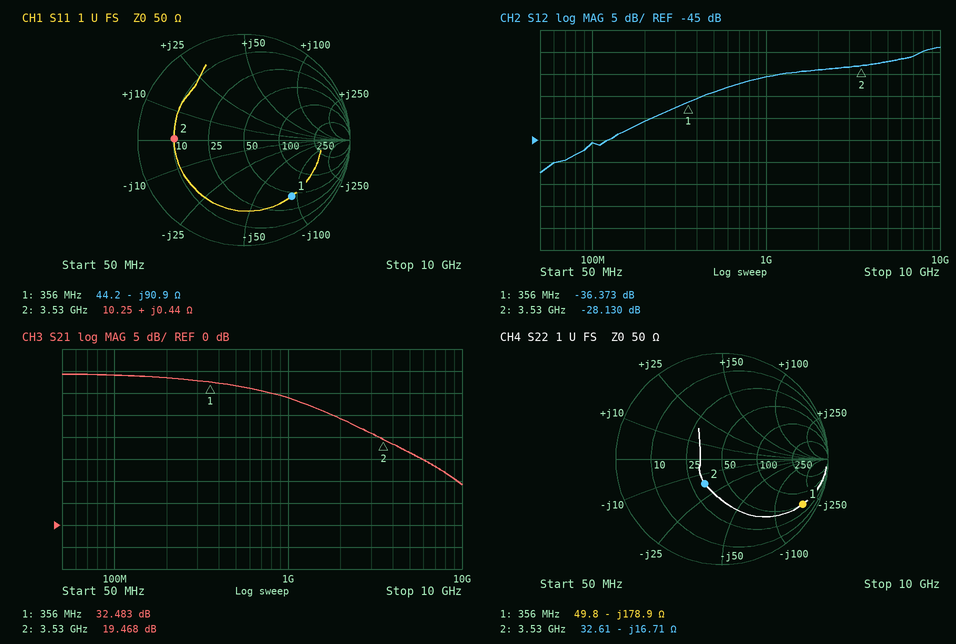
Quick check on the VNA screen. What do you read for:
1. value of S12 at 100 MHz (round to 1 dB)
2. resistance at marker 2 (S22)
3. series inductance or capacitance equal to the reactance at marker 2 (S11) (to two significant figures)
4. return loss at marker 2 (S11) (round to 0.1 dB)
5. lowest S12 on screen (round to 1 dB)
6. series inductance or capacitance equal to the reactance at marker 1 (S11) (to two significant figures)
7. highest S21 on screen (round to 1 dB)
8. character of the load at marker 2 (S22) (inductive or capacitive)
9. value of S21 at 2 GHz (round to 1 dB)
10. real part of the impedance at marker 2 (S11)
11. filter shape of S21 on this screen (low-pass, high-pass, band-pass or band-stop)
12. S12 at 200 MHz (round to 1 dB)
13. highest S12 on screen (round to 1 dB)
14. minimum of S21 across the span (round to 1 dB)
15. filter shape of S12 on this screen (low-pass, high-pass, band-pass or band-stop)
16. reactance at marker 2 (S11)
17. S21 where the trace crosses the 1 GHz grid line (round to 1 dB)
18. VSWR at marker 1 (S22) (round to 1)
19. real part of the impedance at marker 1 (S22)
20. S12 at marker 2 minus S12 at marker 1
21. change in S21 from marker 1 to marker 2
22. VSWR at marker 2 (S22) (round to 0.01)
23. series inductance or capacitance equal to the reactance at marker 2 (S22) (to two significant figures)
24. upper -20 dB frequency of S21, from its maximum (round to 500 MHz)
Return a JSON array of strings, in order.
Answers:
["-46 dB", "32.61 Ω", "20 pH", "3.6 dB", "-52 dB", "4.9 pF", "34 dB", "capacitive", "24 dB", "10.25 Ω", "low-pass", "-41 dB", "-24 dB", "9 dB", "high-pass", "+0.44 Ω", "29 dB", "15", "49.8 Ω", "8.243 dB", "-13.015 dB", "1.80", "2.7 pF", "6.5 GHz"]
